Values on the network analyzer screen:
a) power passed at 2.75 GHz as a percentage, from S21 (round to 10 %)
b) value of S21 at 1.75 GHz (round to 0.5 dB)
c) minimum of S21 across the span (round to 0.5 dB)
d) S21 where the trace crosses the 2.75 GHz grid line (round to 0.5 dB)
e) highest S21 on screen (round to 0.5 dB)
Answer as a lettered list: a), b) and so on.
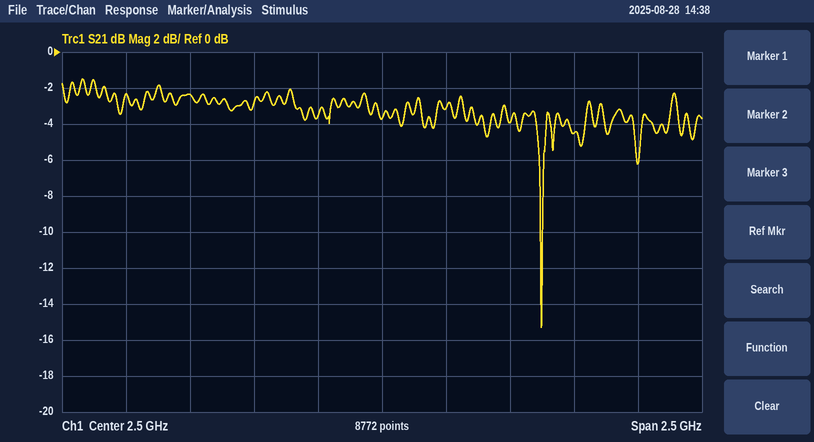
a) 50 %
b) -2.5 dB
c) -15.5 dB
d) -3.0 dB
e) -1.5 dB
